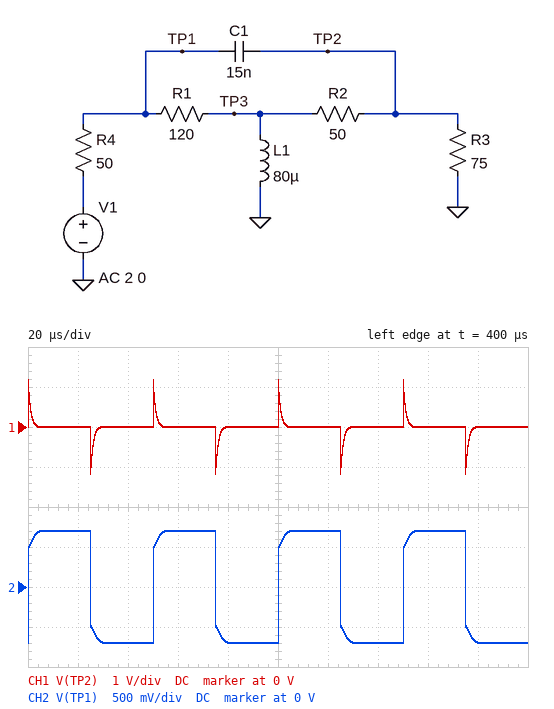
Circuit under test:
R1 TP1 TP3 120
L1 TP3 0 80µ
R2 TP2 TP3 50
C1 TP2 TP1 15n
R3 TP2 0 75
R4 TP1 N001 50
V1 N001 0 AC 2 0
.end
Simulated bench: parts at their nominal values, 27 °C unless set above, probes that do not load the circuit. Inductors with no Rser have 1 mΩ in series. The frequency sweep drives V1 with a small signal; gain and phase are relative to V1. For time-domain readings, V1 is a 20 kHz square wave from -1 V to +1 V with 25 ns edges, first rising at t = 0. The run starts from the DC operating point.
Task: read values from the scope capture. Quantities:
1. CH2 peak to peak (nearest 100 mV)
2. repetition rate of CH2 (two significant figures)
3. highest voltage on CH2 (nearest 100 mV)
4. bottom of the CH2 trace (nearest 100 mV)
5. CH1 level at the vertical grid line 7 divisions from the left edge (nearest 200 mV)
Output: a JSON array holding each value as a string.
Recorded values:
["1.4 V", "20 kHz", "700 mV", "-700 mV", "0 V"]
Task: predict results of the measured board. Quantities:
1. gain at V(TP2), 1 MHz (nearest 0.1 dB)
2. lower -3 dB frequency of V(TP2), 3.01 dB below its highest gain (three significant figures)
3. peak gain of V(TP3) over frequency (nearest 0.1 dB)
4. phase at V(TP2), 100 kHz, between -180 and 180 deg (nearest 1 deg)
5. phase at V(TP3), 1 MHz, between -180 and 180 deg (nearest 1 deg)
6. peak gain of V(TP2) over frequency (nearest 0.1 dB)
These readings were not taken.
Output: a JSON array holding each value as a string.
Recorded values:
["-4.5 dB", "144 kHz", "-4.4 dB", "59 deg", "10 deg", "-4.4 dB"]
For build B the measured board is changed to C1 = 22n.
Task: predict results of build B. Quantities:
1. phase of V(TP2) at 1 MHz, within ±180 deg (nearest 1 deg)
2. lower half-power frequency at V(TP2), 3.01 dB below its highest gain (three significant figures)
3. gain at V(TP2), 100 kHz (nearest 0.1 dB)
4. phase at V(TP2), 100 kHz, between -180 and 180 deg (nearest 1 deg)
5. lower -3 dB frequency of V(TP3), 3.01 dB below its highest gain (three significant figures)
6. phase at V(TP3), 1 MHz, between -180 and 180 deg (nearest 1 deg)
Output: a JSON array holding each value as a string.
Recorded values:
["7 deg", "118 kHz", "-8.3 dB", "52 deg", "152 kHz", "9 deg"]
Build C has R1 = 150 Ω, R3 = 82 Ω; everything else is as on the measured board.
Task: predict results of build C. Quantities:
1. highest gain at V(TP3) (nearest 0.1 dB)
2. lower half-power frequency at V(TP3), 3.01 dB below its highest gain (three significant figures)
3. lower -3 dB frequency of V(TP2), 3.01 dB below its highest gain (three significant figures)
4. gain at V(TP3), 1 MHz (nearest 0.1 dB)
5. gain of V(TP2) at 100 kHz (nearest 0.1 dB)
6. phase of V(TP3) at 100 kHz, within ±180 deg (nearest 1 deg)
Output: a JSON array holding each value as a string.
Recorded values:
["-4.1 dB", "175 kHz", "142 kHz", "-4.2 dB", "-9.2 dB", "72 deg"]
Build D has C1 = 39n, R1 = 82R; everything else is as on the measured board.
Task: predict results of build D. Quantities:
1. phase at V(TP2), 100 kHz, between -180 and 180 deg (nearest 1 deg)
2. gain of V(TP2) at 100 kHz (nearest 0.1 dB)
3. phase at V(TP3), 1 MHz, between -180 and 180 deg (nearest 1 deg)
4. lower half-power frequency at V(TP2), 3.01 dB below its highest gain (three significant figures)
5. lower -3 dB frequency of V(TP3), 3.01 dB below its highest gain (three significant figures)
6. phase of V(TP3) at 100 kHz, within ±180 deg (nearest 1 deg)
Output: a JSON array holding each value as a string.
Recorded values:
["41 deg", "-7.1 dB", "8 deg", "92.4 kHz", "129 kHz", "57 deg"]
